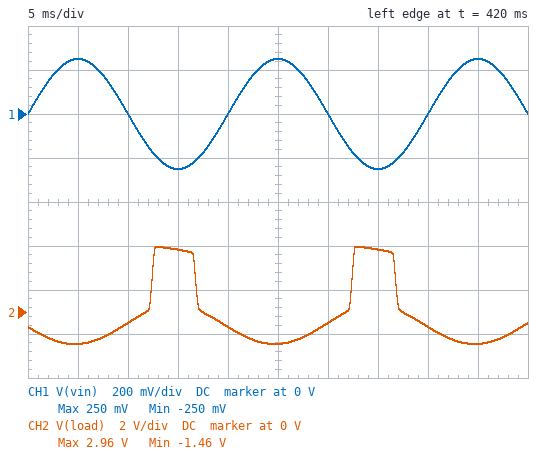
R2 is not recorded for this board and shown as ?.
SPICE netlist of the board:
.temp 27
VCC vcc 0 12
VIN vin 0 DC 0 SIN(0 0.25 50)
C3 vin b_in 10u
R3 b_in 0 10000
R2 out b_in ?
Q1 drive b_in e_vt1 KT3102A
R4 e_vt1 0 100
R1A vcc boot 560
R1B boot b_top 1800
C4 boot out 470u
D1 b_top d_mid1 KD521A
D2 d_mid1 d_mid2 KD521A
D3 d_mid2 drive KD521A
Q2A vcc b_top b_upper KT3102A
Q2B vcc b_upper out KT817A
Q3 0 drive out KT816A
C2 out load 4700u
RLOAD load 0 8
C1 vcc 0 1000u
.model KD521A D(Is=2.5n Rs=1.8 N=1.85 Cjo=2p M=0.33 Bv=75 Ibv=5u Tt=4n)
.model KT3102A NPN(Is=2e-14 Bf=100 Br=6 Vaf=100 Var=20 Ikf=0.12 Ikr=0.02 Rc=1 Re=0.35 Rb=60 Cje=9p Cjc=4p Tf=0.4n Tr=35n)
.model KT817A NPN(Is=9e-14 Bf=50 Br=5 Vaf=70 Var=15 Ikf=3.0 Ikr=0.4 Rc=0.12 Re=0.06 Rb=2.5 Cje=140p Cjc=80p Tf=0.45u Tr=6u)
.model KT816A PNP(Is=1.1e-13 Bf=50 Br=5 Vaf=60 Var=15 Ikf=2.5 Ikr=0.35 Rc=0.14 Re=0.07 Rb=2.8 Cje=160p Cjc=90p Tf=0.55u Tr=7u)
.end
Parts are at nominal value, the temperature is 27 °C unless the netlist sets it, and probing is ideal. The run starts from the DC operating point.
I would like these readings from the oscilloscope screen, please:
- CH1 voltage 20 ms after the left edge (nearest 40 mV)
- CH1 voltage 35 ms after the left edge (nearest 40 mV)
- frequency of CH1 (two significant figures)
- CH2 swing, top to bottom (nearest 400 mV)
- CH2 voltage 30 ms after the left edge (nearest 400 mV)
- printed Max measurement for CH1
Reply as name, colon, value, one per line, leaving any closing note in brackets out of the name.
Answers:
CH1 voltage 20 ms after the left edge: 0 V
CH1 voltage 35 ms after the left edge: -240 mV
frequency of CH1: 50 Hz
CH2 swing, top to bottom: 4.4 V
CH2 voltage 30 ms after the left edge: -400 mV
printed Max measurement for CH1: 250 mV
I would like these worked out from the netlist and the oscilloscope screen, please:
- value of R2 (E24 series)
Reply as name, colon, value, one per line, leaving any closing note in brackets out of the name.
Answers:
value of R2: 62 kΩ
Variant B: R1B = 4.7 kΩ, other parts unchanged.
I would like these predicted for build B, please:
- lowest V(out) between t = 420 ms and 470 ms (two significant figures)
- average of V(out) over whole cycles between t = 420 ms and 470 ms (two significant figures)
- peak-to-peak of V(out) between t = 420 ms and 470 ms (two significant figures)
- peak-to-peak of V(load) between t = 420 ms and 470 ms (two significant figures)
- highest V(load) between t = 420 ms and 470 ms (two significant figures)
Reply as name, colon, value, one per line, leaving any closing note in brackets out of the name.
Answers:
lowest V(out) between t = 420 ms and 470 ms: 6.2 V
average of V(out) over whole cycles between t = 420 ms and 470 ms: 7.7 V
peak-to-peak of V(out) between t = 420 ms and 470 ms: 4.9 V
peak-to-peak of V(load) between t = 420 ms and 470 ms: 5.0 V
highest V(load) between t = 420 ms and 470 ms: 3.5 V
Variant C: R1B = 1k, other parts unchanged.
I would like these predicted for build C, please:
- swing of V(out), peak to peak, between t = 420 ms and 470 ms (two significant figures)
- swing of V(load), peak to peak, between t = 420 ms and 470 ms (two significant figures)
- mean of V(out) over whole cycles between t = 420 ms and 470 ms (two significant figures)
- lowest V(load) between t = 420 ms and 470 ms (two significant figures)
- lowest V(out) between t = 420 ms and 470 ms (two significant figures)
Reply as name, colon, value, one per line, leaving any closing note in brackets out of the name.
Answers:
swing of V(out), peak to peak, between t = 420 ms and 470 ms: 4.0 V
swing of V(load), peak to peak, between t = 420 ms and 470 ms: 4.1 V
mean of V(out) over whole cycles between t = 420 ms and 470 ms: 8.6 V
lowest V(load) between t = 420 ms and 470 ms: -1.4 V
lowest V(out) between t = 420 ms and 470 ms: 7.2 V
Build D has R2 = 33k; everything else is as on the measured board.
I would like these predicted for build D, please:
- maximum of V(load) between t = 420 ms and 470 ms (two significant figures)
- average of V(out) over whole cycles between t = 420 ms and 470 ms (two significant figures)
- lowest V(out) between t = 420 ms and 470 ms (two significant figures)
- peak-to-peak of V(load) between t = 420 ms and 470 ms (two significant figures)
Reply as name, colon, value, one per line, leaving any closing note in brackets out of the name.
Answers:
maximum of V(load) between t = 420 ms and 470 ms: 5.1 V
average of V(out) over whole cycles between t = 420 ms and 470 ms: 5.9 V
lowest V(out) between t = 420 ms and 470 ms: 4.4 V
peak-to-peak of V(load) between t = 420 ms and 470 ms: 6.6 V
